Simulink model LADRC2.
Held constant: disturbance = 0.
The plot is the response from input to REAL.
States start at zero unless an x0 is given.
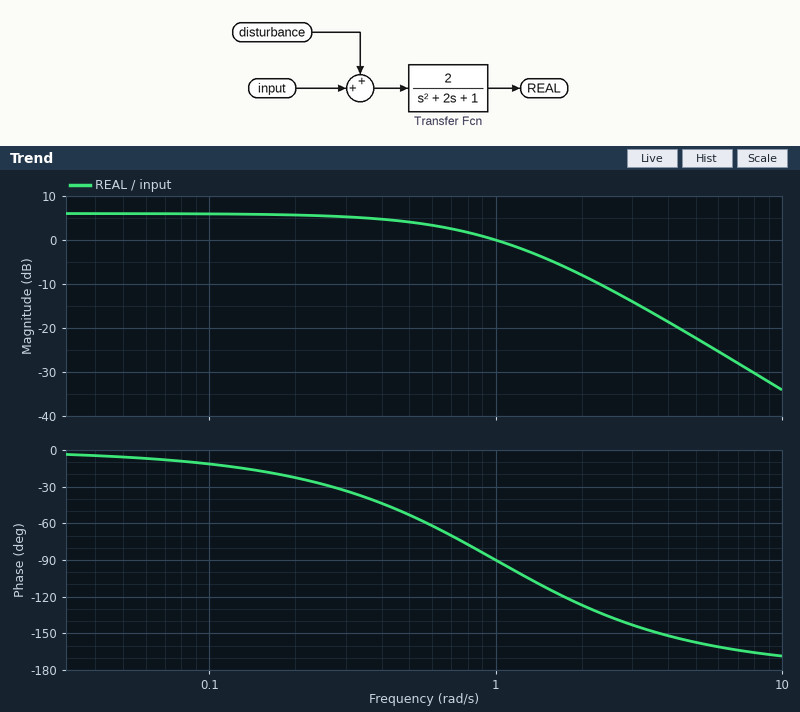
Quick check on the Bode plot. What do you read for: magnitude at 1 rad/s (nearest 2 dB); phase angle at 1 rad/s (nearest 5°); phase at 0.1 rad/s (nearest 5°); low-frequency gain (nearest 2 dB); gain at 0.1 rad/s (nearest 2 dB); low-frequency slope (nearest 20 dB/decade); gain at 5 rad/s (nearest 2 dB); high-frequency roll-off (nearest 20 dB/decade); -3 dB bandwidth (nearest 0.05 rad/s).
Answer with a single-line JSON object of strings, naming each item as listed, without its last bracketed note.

{"magnitude at 1 rad/s": "0 dB", "phase angle at 1 rad/s": "-90°", "phase at 0.1 rad/s": "-10°", "low-frequency gain": "6 dB", "gain at 0.1 rad/s": "6 dB", "low-frequency slope": "0 dB/decade", "gain at 5 rad/s": "-22 dB", "high-frequency roll-off": "-40 dB/decade", "-3 dB bandwidth": "0.65 rad/s"}
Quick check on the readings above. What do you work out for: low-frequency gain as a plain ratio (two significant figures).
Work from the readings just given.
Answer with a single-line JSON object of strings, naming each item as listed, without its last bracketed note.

{"low-frequency gain as a plain ratio": "2.0"}
